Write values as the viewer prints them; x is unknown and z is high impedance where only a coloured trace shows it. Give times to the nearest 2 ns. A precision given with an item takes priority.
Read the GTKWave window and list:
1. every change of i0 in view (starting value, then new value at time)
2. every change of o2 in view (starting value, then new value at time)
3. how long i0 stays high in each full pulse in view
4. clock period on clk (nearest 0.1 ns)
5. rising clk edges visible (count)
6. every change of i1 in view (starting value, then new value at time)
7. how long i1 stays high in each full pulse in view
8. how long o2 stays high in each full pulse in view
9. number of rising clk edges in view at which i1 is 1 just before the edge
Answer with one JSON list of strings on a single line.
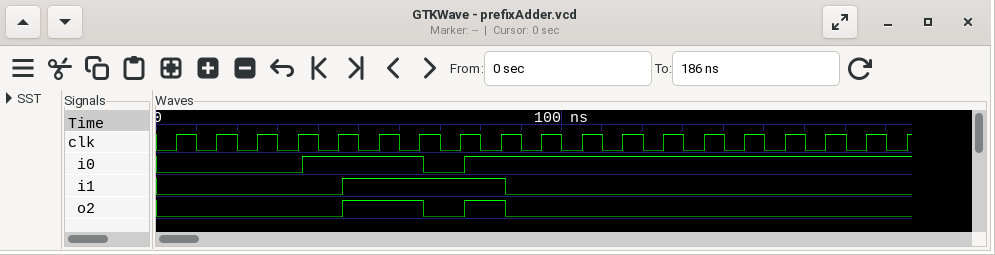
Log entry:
["0, 1 at 36 ns, 0 at 66 ns, 1 at 76 ns", "0, 1 at 46 ns, 0 at 66 ns, 1 at 76 ns, 0 at 86 ns", "30 ns", "10 ns", "19", "0, 1 at 46 ns, 0 at 86 ns", "40 ns", "20 ns, 10 ns", "4"]
